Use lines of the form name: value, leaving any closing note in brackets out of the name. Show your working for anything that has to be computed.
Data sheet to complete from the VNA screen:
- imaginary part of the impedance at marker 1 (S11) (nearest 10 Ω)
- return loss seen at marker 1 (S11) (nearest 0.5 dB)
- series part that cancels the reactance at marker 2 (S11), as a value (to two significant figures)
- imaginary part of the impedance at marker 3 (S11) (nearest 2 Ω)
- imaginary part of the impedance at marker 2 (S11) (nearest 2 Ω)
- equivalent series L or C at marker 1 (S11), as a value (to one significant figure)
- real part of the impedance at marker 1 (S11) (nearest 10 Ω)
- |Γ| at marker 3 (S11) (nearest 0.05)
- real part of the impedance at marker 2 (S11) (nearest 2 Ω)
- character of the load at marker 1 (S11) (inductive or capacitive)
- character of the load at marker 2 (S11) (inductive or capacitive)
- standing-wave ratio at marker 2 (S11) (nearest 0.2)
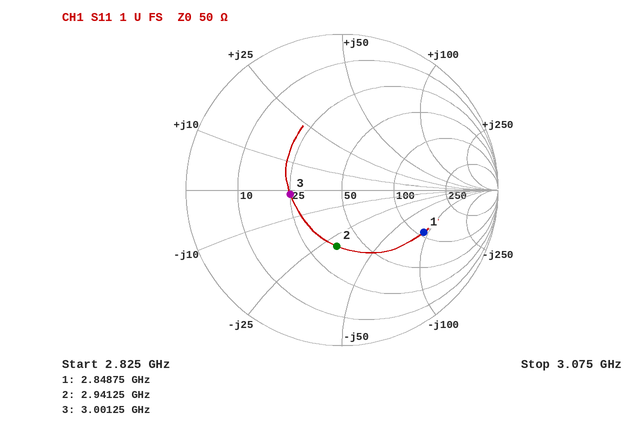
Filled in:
imaginary part of the impedance at marker 1 (S11): -90 Ω
return loss seen at marker 1 (S11): 4.5 dB
series part that cancels the reactance at marker 2 (S11), as a value: L = 30 Ω/(2π × 2.94125 GHz) ≈ 1.6 nH
imaginary part of the impedance at marker 3 (S11): -2 Ω
imaginary part of the impedance at marker 2 (S11): -30 Ω
equivalent series L or C at marker 1 (S11), as a value: C = 1/(2π × 2.84875 GHz × 90 Ω) ≈ 621 fF, so 600 fF to one significant figure
real part of the impedance at marker 1 (S11): 110 Ω
|Γ| at marker 3 (S11): 0.35
real part of the impedance at marker 2 (S11): 36 Ω
character of the load at marker 1 (S11): capacitive
character of the load at marker 2 (S11): capacitive
standing-wave ratio at marker 2 (S11): 2.2
